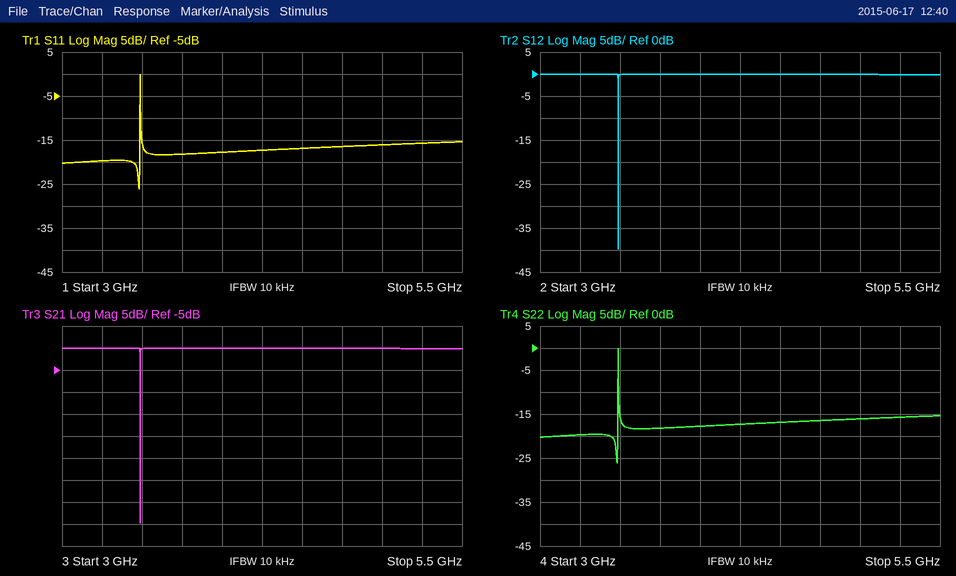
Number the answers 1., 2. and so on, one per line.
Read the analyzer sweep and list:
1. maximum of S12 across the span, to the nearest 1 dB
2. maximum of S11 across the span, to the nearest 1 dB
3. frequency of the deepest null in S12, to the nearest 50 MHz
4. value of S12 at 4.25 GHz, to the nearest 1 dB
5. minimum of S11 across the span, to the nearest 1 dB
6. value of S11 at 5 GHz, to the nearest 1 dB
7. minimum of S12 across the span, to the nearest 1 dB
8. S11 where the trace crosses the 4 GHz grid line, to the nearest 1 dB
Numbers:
1. 0 dB
2. 0 dB
3. 3.50 GHz
4. 0 dB
5. -26 dB
6. -16 dB
7. -40 dB
8. -18 dB
